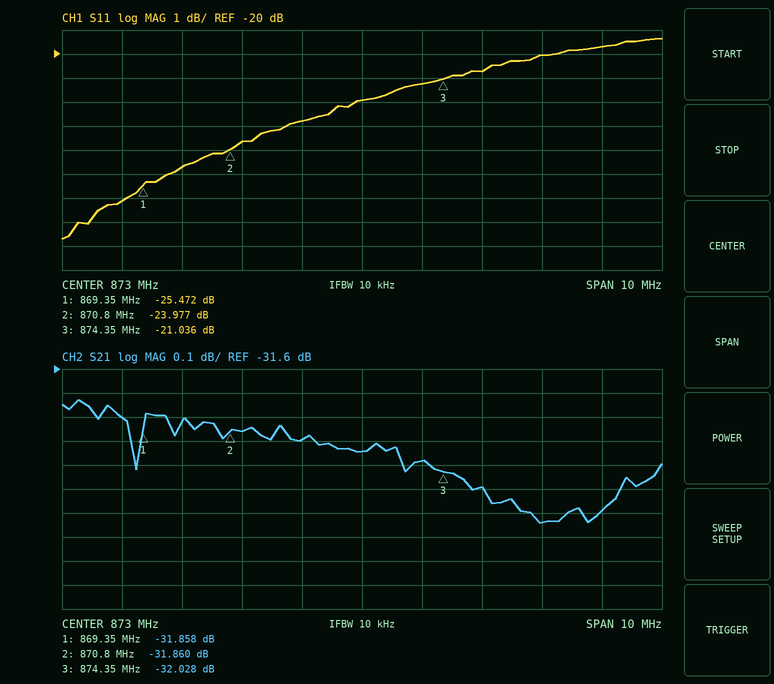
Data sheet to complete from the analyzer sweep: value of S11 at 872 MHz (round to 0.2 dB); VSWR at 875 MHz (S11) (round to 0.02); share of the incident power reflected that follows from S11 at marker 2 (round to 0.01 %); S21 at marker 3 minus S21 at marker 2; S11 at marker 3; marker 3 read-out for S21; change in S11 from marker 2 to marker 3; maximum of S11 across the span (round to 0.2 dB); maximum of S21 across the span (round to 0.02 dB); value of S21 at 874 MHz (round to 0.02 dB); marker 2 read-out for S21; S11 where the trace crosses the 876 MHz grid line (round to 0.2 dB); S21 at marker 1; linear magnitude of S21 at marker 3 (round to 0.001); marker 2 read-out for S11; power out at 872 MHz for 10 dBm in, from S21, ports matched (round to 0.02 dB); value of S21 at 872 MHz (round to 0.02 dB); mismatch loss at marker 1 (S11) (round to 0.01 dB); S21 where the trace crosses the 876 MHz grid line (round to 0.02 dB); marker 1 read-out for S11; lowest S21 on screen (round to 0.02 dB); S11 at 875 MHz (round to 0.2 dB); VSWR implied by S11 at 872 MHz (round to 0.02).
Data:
-22.8 dB
1.20
0.40 %
-0.168 dB
-21.036 dB
-32.028 dB
2.941 dB
-19.4 dB
-31.72 dB
-31.98 dB
-31.860 dB
-20.0 dB
-31.858 dB
0.025
-23.977 dB
-21.90 dBm
-31.90 dB
0.01 dB
-32.24 dB
-25.472 dB
-32.24 dB
-20.8 dB
1.16
